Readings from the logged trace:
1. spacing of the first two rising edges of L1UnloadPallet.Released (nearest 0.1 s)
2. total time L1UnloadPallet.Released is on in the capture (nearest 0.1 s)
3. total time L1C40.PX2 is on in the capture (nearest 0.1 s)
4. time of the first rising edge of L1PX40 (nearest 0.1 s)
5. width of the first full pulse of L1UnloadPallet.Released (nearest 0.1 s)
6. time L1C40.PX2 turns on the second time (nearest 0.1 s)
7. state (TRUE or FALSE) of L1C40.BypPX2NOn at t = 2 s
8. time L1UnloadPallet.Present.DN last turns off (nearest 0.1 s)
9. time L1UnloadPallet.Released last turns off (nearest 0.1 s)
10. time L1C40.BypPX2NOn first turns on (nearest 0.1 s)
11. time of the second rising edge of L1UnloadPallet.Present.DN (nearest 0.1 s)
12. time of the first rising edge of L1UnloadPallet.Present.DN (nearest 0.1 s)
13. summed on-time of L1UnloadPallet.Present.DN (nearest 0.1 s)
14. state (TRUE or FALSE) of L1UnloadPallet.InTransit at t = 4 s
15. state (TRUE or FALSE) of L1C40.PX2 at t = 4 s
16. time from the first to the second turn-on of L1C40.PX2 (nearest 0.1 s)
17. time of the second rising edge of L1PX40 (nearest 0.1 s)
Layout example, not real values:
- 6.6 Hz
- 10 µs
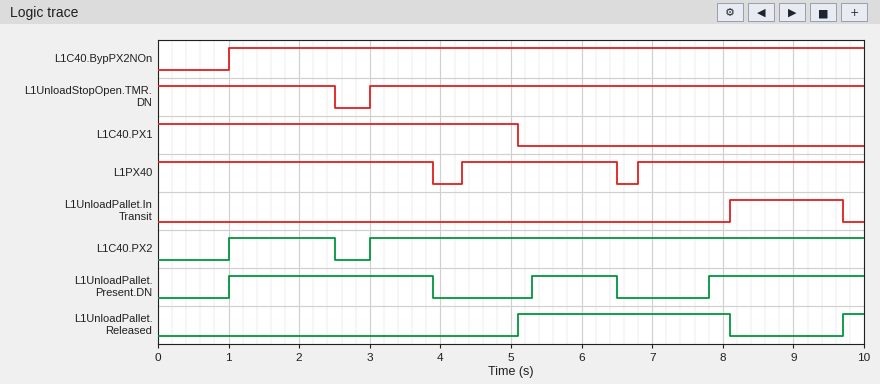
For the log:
- 4.6 s
- 3.3 s
- 8.5 s
- 4.3 s
- 3.0 s
- 3.0 s
- TRUE
- 6.5 s
- 8.1 s
- 1.0 s
- 5.3 s
- 1.0 s
- 6.3 s
- FALSE
- TRUE
- 2.0 s
- 6.8 s
